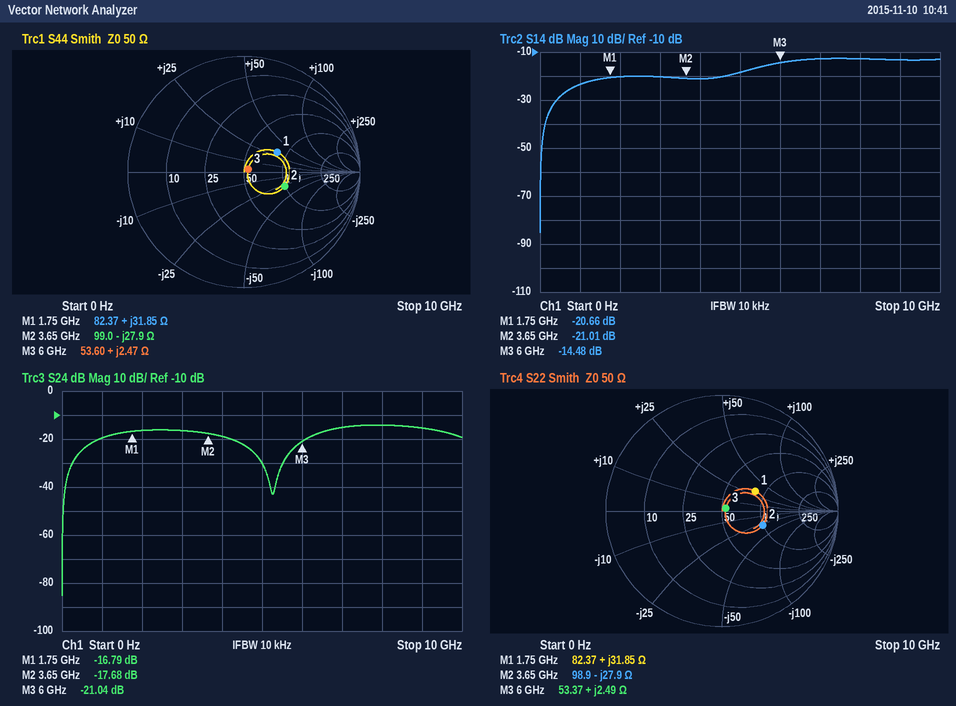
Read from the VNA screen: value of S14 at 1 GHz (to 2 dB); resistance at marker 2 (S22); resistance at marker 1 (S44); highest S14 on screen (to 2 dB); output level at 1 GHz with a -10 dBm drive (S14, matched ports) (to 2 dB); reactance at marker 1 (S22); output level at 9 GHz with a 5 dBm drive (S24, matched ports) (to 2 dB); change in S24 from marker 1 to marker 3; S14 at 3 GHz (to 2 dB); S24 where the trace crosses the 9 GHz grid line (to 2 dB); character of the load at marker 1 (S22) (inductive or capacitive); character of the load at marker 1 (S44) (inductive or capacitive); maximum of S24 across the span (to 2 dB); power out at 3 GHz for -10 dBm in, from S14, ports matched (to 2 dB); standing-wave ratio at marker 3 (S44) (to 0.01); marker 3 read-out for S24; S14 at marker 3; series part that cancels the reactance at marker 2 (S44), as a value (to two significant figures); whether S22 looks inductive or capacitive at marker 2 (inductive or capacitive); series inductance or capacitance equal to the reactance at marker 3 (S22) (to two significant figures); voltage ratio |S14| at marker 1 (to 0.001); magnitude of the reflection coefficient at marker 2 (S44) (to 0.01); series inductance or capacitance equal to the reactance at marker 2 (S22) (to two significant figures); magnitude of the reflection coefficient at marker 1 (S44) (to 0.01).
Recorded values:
-24 dB
98.9 Ω
82.37 Ω
-12 dB
-34 dBm
+31.85 Ω
-10 dBm
-4.25 dB
-20 dB
-16 dB
inductive
inductive
-14 dB
-30 dBm
1.09
-21.04 dB
-14.48 dB
1.2 nH
capacitive
66 pH
0.093
0.37
1.6 pF
0.33
